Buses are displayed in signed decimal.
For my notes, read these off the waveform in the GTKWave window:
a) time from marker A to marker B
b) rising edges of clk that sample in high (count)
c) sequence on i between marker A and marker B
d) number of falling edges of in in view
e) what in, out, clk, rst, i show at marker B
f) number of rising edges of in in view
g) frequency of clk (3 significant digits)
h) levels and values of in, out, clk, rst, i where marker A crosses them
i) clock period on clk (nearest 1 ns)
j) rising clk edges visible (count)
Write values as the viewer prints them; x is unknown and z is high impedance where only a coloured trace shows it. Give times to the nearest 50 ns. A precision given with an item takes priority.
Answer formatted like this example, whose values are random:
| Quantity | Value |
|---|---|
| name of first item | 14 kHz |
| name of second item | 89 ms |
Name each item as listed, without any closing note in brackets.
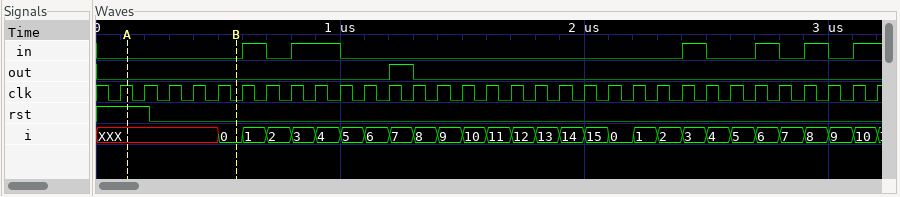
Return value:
| Quantity | Value |
|---|---|
| time from marker A to marker B | 450 ns |
| rising edges of clk that sample in high | 7 |
| sequence on i between marker A and marker B | XXX, 0 |
| number of falling edges of in in view | 5 |
| what in, out, clk, rst, i show at marker B | in=0, out=0, clk=0, rst=0, i=0 |
| number of rising edges of in in view | 6 |
| frequency of clk | 10.0 MHz |
| levels and values of in, out, clk, rst, i where marker A crosses them | in=0, out=0, clk=1, rst=1, i=XXX |
| clock period on clk | 100 ns |
| rising clk edges visible | 32 |
